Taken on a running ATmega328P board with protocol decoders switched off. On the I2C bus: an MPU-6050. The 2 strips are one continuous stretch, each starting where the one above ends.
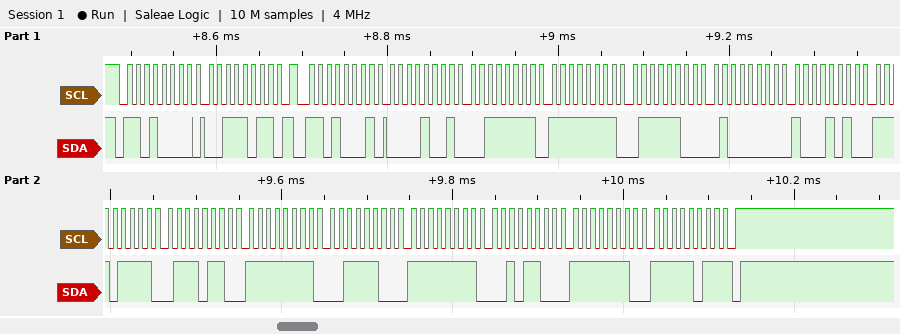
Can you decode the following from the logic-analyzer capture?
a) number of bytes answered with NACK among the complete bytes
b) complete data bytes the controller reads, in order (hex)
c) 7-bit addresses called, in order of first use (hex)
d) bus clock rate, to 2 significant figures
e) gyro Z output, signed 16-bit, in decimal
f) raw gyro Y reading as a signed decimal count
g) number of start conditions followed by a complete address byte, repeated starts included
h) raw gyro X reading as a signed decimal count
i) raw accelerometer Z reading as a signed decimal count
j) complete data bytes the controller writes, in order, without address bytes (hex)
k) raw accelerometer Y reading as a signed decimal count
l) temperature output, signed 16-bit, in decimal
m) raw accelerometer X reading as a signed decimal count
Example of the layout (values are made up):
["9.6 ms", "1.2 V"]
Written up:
["1", "09 3F FF 7C 40 8A EF 76 FF 3C FF 2C FE FB", "0x68", "100 kHz", "-261", "-212", "2", "-196", "16522", "3B", "-132", "-4234", "2367"]
